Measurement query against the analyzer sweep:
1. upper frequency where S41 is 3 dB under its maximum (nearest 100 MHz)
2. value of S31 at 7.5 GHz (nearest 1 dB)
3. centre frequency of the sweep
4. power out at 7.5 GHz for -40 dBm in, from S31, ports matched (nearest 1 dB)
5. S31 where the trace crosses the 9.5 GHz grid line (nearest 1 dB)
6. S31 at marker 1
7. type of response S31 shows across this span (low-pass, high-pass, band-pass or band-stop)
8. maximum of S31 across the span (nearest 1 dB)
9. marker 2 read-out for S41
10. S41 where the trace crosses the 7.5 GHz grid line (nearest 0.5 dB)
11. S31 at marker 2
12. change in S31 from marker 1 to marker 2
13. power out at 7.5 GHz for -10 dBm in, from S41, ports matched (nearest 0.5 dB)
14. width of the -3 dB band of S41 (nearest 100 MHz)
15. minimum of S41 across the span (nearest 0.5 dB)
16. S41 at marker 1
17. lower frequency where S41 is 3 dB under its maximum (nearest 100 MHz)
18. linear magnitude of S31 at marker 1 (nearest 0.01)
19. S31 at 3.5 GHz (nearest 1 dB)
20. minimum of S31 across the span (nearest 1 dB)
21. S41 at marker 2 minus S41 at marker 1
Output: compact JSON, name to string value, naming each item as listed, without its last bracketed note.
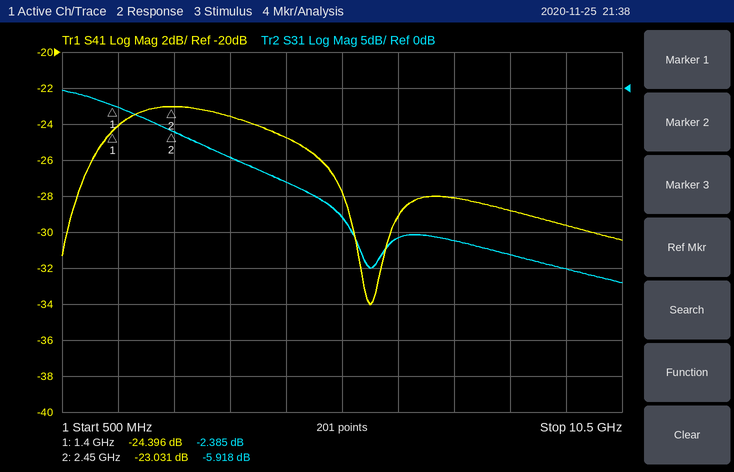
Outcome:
{"upper frequency where S41 is 3 dB under its maximum": "5.1 GHz", "value of S31 at 7.5 GHz": "-21 dB", "centre frequency of the sweep": "5.5 GHz", "power out at 7.5 GHz for -40 dBm in, from S31, ports matched": "-61 dBm", "S31 where the trace crosses the 9.5 GHz grid line": "-25 dB", "S31 at marker 1": "-2.385 dB", "type of response S31 shows across this span": "low-pass", "maximum of S31 across the span": "0 dB", "marker 2 read-out for S41": "-23.031 dB", "S41 where the trace crosses the 7.5 GHz grid line": "-28.0 dB", "S31 at marker 2": "-5.918 dB", "change in S31 from marker 1 to marker 2": "-3.533 dB", "power out at 7.5 GHz for -10 dBm in, from S41, ports matched": "-38.0 dBm", "width of the -3 dB band of S41": "4.1 GHz", "minimum of S41 across the span": "-34.0 dB", "S41 at marker 1": "-24.396 dB", "lower frequency where S41 is 3 dB under its maximum": "1.0 GHz", "linear magnitude of S31 at marker 1": "0.76", "S31 at 3.5 GHz": "-10 dB", "minimum of S31 across the span": "-27 dB", "S41 at marker 2 minus S41 at marker 1": "1.365 dB"}
